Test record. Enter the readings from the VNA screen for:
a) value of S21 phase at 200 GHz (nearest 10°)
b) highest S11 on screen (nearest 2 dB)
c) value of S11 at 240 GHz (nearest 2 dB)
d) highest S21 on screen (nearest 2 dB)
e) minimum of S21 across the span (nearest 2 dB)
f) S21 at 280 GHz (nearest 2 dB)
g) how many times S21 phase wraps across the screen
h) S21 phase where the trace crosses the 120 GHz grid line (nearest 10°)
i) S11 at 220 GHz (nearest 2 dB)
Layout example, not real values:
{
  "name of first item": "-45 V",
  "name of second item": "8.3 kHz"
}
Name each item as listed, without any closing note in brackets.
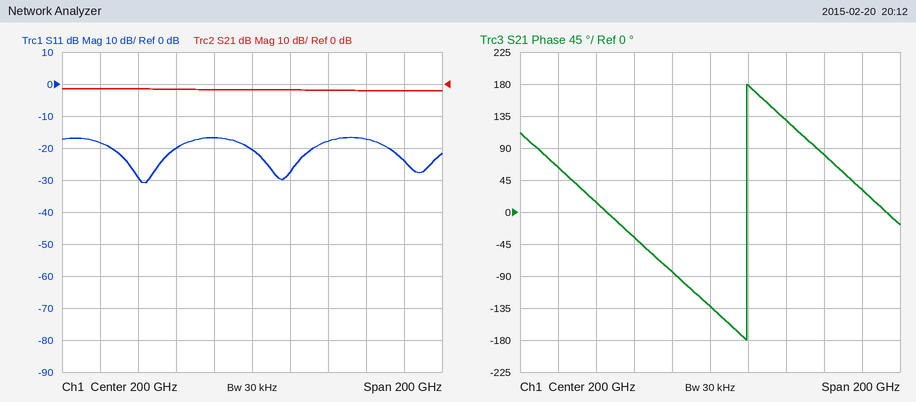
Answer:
{
  "value of S21 phase at 200 GHz": "-130°",
  "highest S11 on screen": "-16 dB",
  "value of S11 at 240 GHz": "-18 dB",
  "highest S21 on screen": "-2 dB",
  "minimum of S21 across the span": "-2 dB",
  "S21 at 280 GHz": "-2 dB",
  "how many times S21 phase wraps across the screen": "1",
  "S21 phase where the trace crosses the 120 GHz grid line": "60°",
  "S11 at 220 GHz": "-28 dB"
}
